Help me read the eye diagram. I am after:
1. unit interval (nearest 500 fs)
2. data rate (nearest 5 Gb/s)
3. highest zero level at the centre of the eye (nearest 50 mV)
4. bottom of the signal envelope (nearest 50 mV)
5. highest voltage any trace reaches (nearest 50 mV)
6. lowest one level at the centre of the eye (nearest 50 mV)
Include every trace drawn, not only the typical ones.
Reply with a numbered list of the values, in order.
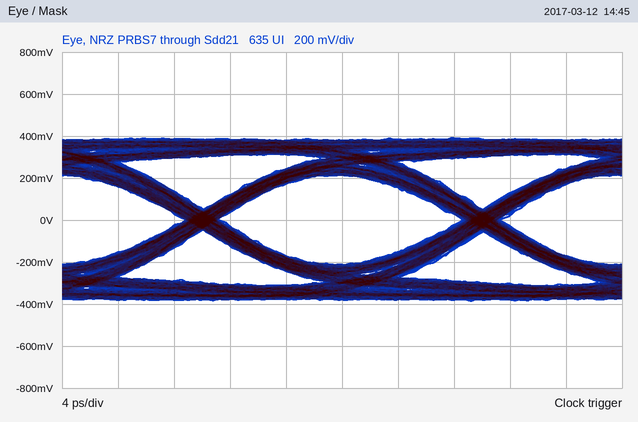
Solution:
1. 20.0 ps
2. 50 Gb/s
3. -200 mV
4. -400 mV
5. 400 mV
6. 200 mV
